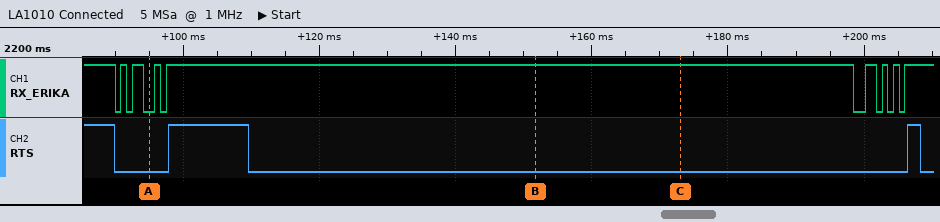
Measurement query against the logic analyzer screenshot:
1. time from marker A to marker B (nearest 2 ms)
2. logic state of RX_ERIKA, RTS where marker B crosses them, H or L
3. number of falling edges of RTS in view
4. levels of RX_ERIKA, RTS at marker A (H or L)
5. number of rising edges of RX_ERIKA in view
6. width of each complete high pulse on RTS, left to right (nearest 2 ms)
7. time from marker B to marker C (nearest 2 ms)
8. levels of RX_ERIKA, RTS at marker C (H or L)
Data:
56 ms
RX_ERIKA=H, RTS=L
3
RX_ERIKA=L, RTS=L
8
12 ms, 2 ms
22 ms
RX_ERIKA=H, RTS=L
